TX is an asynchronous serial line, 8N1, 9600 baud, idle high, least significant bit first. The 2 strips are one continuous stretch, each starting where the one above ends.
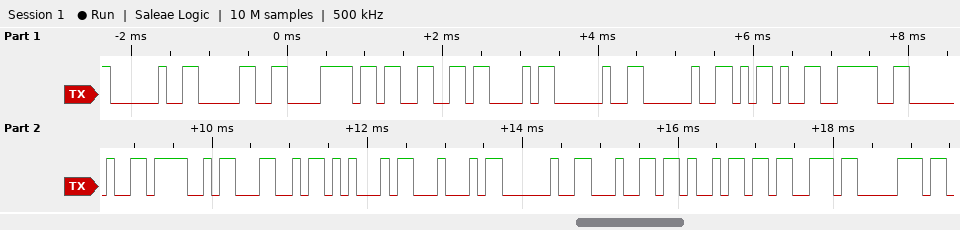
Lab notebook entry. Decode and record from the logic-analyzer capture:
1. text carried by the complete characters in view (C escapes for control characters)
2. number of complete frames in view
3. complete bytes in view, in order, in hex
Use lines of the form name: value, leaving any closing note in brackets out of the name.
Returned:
text carried by the complete characters in view: " 0x3C  -> OLED disp"
number of complete frames in view: 19
complete bytes in view, in order, in hex: 0x20 0x30 0x78 0x33 0x43 0x20 0x20 0x2D 0x3E 0x20 0x4F 0x4C 0x45 0x44 0x20 0x64 0x69 0x73 0x70
